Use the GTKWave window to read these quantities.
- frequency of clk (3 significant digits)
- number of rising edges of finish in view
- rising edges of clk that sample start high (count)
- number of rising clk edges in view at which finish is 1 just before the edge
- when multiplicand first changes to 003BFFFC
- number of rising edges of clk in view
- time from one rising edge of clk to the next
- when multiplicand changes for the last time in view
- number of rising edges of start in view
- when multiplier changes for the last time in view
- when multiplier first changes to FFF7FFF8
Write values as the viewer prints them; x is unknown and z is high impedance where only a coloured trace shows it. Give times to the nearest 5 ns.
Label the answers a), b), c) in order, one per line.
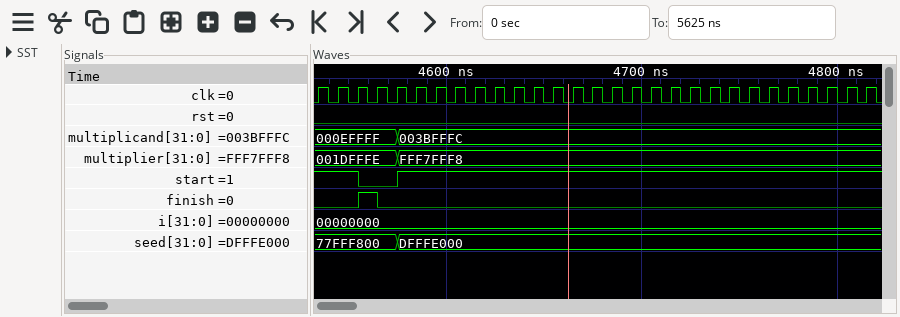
a) 100 MHz
b) 1
c) 27
d) 1
e) 4575 ns
f) 29
g) 10 ns
h) 4575 ns
i) 1
j) 4575 ns
k) 4575 ns
